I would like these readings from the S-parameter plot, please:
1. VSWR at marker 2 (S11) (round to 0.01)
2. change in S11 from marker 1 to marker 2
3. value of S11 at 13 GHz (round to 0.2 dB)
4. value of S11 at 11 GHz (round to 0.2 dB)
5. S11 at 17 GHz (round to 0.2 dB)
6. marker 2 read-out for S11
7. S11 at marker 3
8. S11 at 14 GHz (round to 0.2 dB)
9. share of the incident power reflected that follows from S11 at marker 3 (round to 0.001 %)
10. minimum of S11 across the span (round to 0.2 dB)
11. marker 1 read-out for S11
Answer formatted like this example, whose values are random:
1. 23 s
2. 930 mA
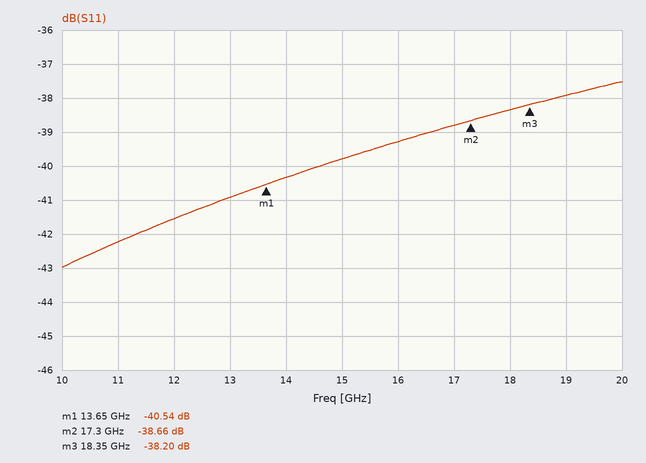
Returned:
1. 1.02
2. 1.88 dB
3. -41.0 dB
4. -42.2 dB
5. -38.8 dB
6. -38.66 dB
7. -38.20 dB
8. -40.4 dB
9. 0.015 %
10. -43.0 dB
11. -40.54 dB
